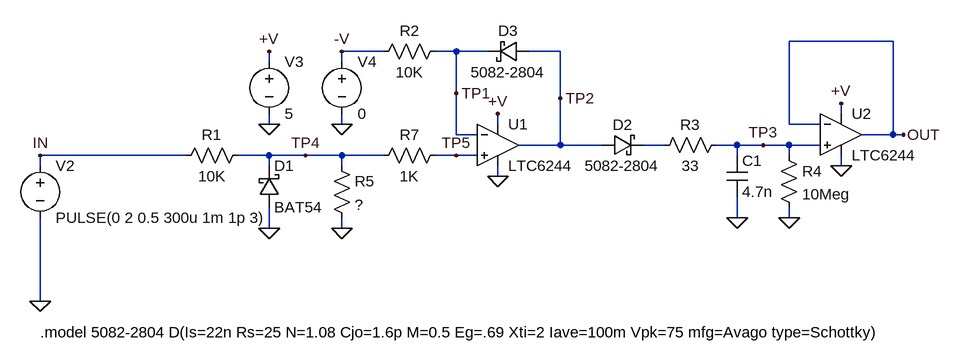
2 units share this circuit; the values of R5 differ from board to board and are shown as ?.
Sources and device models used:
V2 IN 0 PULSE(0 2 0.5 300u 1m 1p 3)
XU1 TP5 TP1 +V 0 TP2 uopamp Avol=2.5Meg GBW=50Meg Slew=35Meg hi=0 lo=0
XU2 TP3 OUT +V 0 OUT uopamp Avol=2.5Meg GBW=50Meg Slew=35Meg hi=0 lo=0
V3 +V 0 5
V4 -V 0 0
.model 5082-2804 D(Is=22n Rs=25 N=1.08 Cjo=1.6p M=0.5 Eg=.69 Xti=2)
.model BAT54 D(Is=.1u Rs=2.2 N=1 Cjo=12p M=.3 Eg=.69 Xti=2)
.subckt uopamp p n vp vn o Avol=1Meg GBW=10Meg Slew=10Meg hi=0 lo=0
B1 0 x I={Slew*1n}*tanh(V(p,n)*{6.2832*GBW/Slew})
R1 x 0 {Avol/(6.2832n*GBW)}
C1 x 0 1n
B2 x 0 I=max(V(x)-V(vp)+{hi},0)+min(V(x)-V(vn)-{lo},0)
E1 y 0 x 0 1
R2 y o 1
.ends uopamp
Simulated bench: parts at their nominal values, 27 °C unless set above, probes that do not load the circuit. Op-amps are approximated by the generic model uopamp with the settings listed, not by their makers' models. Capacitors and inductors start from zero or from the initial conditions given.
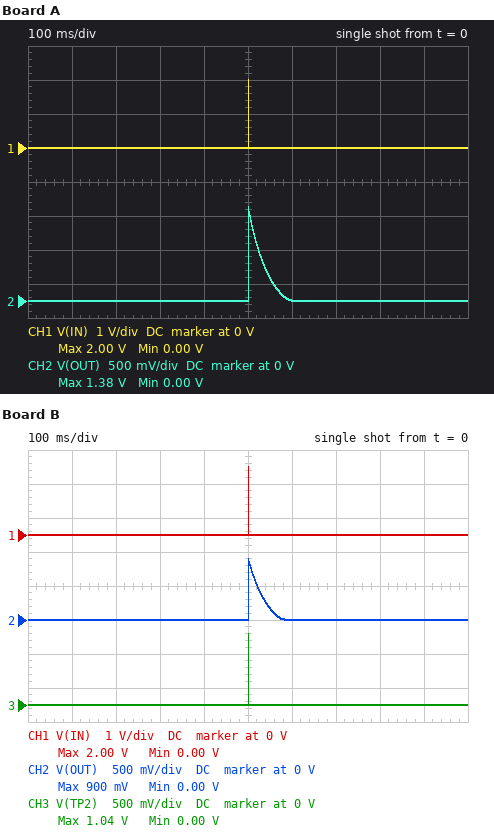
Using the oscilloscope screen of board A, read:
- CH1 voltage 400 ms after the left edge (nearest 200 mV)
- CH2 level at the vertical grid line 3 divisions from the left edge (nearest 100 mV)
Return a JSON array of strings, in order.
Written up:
["0 V", "0 V"]
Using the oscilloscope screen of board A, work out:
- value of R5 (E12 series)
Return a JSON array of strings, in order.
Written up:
["18 kΩ"]
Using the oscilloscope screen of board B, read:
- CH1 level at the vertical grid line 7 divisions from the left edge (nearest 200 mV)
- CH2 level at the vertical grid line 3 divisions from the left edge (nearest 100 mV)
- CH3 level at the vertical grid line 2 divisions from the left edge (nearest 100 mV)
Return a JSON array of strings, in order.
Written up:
["0 V", "0 V", "0 V"]
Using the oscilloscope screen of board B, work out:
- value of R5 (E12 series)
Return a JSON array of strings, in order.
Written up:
["6.8 kΩ"]
